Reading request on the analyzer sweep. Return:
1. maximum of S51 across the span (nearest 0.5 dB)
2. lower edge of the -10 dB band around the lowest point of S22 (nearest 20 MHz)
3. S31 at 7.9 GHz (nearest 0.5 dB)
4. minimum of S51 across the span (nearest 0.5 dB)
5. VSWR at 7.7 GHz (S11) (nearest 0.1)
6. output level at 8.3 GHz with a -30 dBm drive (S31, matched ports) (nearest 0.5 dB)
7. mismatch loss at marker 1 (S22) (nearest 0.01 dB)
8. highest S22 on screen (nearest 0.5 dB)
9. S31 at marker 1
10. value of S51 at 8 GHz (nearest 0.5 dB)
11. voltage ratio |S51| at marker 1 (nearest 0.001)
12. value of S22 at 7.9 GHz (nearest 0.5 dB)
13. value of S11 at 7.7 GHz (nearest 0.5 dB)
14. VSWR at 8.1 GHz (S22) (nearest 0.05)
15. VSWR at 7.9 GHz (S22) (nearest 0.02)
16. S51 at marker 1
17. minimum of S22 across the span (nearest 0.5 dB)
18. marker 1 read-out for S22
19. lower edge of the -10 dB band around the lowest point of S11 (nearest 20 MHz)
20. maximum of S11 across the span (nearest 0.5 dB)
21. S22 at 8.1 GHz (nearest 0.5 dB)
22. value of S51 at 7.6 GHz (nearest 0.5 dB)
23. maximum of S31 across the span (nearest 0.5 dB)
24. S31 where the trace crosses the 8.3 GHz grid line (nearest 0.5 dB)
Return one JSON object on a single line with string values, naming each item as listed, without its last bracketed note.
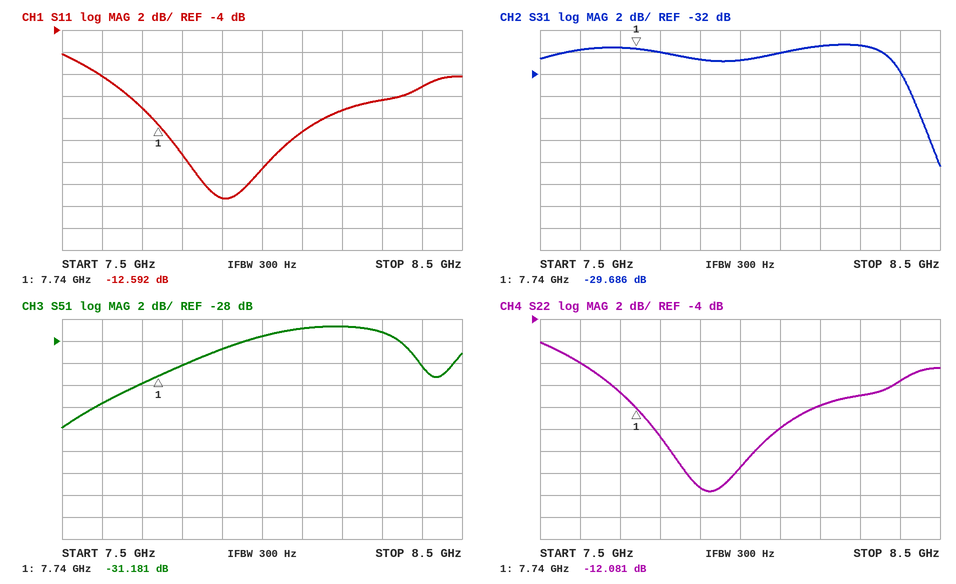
{"maximum of S51 across the span": "-26.5 dB", "lower edge of the -10 dB band around the lowest point of S22": "7.68 GHz", "S31 at 7.9 GHz": "-30.5 dB", "minimum of S51 across the span": "-36.0 dB", "VSWR at 7.7 GHz (S11)": "1.8", "output level at 8.3 GHz with a -30 dBm drive (S31, matched ports)": "-59.5 dBm", "mismatch loss at marker 1 (S22)": "0.28 dB", "highest S22 on screen": "-6.0 dB", "S31 at marker 1": "-29.686 dB", "value of S51 at 8 GHz": "-27.5 dB", "voltage ratio |S51| at marker 1": "0.028", "value of S22 at 7.9 GHz": "-19.5 dB", "value of S11 at 7.7 GHz": "-11.0 dB", "VSWR at 8.1 GHz (S22)": "1.50", "VSWR at 7.9 GHz (S22)": "1.24", "S51 at marker 1": "-31.181 dB", "minimum of S22 across the span": "-19.5 dB", "marker 1 read-out for S22": "-12.081 dB", "lower edge of the -10 dB band around the lowest point of S11": "7.66 GHz", "maximum of S11 across the span": "-6.0 dB", "S22 at 8.1 GHz": "-14.0 dB", "value of S51 at 7.6 GHz": "-33.5 dB", "maximum of S31 across the span": "-29.5 dB", "S31 where the trace crosses the 8.3 GHz grid line": "-29.5 dB"}
